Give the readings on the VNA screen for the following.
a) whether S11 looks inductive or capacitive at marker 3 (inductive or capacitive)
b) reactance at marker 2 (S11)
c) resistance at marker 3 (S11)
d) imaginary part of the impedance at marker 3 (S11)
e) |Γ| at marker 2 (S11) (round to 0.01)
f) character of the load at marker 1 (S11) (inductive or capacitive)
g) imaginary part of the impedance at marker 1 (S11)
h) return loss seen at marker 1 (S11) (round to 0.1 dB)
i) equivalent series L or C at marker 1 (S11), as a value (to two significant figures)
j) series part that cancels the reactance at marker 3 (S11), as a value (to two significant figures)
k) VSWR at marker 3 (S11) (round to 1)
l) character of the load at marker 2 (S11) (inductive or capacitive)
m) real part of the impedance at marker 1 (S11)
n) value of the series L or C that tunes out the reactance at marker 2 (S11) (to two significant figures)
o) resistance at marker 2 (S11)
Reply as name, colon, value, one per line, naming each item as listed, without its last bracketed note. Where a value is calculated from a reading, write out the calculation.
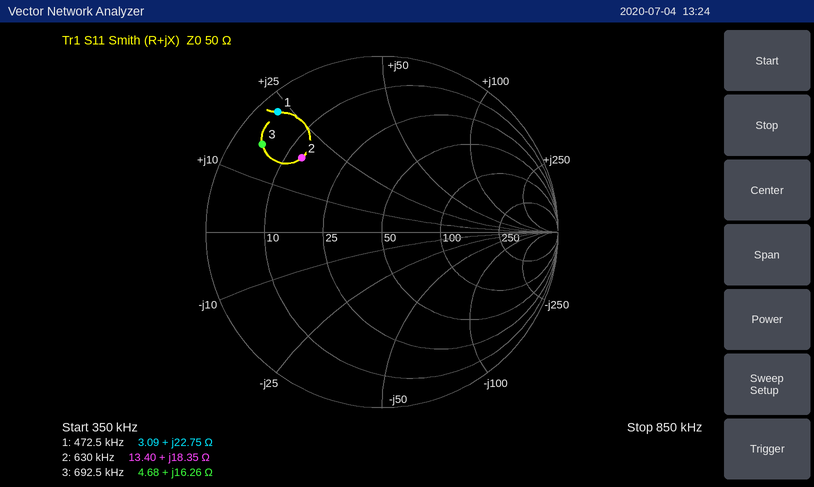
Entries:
whether S11 looks inductive or capacitive at marker 3: inductive
reactance at marker 2: +18.35 Ω
resistance at marker 3: 4.68 Ω
imaginary part of the impedance at marker 3: +16.26 Ω
|Γ| at marker 2 (S11): 0.62
character of the load at marker 1 (S11): inductive
imaginary part of the impedance at marker 1: +22.75 Ω
return loss seen at marker 1 (S11): 0.9 dB
equivalent series L or C at marker 1 (S11), as a value: L = 22.75 Ω/(2π × 472.5 kHz) ≈ 7.7 µH
series part that cancels the reactance at marker 3 (S11), as a value: C = 1/(2π × 692.5 kHz × 16.26 Ω) ≈ 14 nF
VSWR at marker 3 (S11): 12
character of the load at marker 2 (S11): inductive
real part of the impedance at marker 1: 3.09 Ω
value of the series L or C that tunes out the reactance at marker 2 (S11): C = 1/(2π × 630 kHz × 18.35 Ω) ≈ 14 nF
resistance at marker 2: 13.40 Ω
